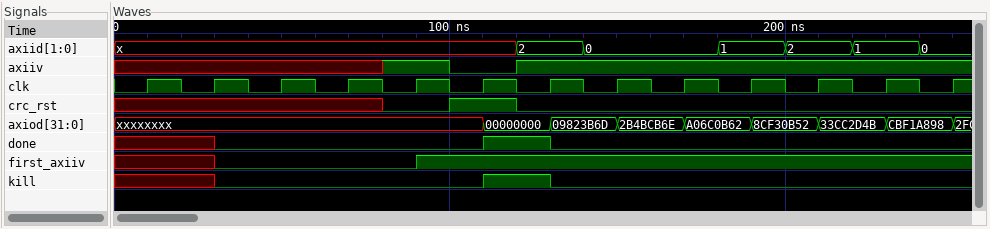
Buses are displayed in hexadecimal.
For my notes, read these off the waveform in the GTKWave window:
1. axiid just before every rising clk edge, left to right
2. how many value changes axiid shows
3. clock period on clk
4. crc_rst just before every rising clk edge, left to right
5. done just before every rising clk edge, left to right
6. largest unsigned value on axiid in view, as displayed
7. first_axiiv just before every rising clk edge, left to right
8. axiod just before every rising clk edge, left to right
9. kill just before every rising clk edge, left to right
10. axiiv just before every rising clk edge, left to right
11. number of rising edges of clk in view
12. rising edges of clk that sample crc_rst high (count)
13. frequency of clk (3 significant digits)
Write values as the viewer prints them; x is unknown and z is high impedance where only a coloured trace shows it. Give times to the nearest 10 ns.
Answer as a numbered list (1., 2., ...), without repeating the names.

1. x, x, x, x, x, x, 2, 0, 0, 1, 2, 1, 0
2. 6
3. 20 ns
4. x x x x 0 1 0 0 0 0 0 0 0
5. x x 0 0 0 0 1 0 0 0 0 0 0
6. 2
7. x x 0 0 0 1 1 1 1 1 1 1 1
8. xxxxxxxx, xxxxxxxx, xxxxxxxx, xxxxxxxx, xxxxxxxx, xxxxxxxx, 00000000, 09823B6D, 2B4BCB6E, A06C0B62, 8CF30B52, 33CC2D4B, CBF1A898
9. x x 0 0 0 0 1 0 0 0 0 0 0
10. x x x x 1 0 1 1 1 1 1 1 1
11. 13
12. 1
13. 50.0 MHz
